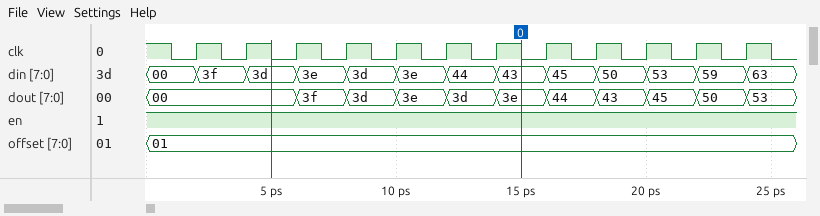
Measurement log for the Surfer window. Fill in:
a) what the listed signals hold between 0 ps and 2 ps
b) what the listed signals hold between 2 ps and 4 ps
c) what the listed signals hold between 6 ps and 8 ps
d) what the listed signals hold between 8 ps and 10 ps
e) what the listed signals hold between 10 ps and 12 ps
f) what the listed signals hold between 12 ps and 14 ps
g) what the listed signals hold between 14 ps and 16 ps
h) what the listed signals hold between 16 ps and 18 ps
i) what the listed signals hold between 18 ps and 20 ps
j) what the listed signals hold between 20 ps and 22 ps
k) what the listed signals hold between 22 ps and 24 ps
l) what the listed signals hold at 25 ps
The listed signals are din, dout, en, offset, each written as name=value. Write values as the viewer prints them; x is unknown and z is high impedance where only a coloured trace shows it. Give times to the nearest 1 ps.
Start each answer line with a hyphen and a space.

- din=00, dout=00, en=1, offset=01
- din=3f, dout=00, en=1, offset=01
- din=3e, dout=3f, en=1, offset=01
- din=3d, dout=3d, en=1, offset=01
- din=3e, dout=3e, en=1, offset=01
- din=44, dout=3d, en=1, offset=01
- din=43, dout=3e, en=1, offset=01
- din=45, dout=44, en=1, offset=01
- din=50, dout=43, en=1, offset=01
- din=53, dout=45, en=1, offset=01
- din=59, dout=50, en=1, offset=01
- din=63, dout=53, en=1, offset=01
